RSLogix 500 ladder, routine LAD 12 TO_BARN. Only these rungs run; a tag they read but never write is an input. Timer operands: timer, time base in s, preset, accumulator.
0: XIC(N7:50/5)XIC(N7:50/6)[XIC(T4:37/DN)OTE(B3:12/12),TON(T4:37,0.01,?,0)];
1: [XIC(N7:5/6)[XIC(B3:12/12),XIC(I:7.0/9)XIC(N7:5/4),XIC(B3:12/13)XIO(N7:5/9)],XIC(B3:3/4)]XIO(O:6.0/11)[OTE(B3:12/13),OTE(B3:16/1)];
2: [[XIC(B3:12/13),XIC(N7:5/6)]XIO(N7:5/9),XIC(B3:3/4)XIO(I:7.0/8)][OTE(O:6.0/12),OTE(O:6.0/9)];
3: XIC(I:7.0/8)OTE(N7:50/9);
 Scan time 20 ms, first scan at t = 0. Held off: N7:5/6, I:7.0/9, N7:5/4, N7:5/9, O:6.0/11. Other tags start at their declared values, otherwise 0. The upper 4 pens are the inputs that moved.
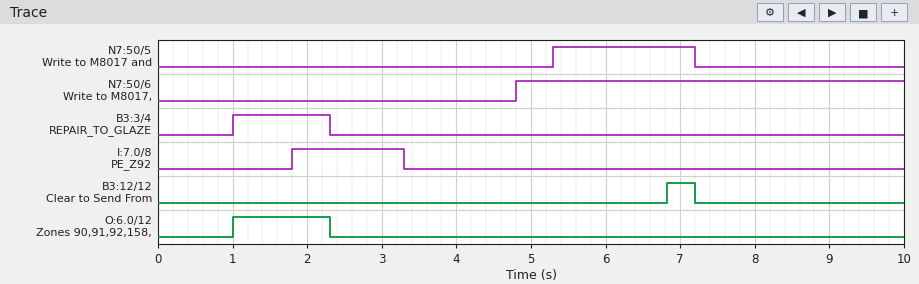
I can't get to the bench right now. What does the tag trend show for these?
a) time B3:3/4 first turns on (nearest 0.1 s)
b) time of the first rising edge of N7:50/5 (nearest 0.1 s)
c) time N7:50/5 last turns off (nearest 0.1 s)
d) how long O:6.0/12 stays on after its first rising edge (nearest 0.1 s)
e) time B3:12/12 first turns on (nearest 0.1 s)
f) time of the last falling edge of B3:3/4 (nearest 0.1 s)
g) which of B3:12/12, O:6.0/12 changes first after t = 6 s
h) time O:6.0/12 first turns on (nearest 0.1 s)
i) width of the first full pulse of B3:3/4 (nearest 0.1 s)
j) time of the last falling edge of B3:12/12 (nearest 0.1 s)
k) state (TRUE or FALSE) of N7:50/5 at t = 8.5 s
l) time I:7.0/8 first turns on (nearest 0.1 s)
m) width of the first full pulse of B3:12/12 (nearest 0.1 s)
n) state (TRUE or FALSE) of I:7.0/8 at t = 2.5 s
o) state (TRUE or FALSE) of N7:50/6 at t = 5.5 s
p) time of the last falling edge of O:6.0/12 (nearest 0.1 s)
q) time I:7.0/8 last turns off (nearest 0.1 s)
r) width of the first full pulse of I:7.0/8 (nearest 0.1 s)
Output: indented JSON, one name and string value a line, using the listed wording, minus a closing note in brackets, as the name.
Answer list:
{
  "time B3:3/4 first turns on": "1.0 s",
  "time of the first rising edge of N7:50/5": "5.3 s",
  "time N7:50/5 last turns off": "7.2 s",
  "how long O:6.0/12 stays on after its first rising edge": "1.3 s",
  "time B3:12/12 first turns on": "6.8 s",
  "time of the last falling edge of B3:3/4": "2.3 s",
  "which of B3:12/12, O:6.0/12 changes first after t = 6 s": "B3:12/12",
  "time O:6.0/12 first turns on": "1.0 s",
  "width of the first full pulse of B3:3/4": "1.3 s",
  "time of the last falling edge of B3:12/12": "7.2 s",
  "state (TRUE or FALSE) of N7:50/5 at t = 8.5 s": "FALSE",
  "time I:7.0/8 first turns on": "1.8 s",
  "width of the first full pulse of B3:12/12": "0.4 s",
  "state (TRUE or FALSE) of I:7.0/8 at t = 2.5 s": "TRUE",
  "state (TRUE or FALSE) of N7:50/6 at t = 5.5 s": "TRUE",
  "time of the last falling edge of O:6.0/12": "2.3 s",
  "time I:7.0/8 last turns off": "3.3 s",
  "width of the first full pulse of I:7.0/8": "1.5 s"
}
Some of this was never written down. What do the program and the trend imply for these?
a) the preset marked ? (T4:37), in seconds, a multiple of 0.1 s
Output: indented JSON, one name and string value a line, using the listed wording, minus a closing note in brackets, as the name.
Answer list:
{
  "the preset marked ? (T4:37), in seconds, a multiple of 0.1 s": "1.5 s"
}
